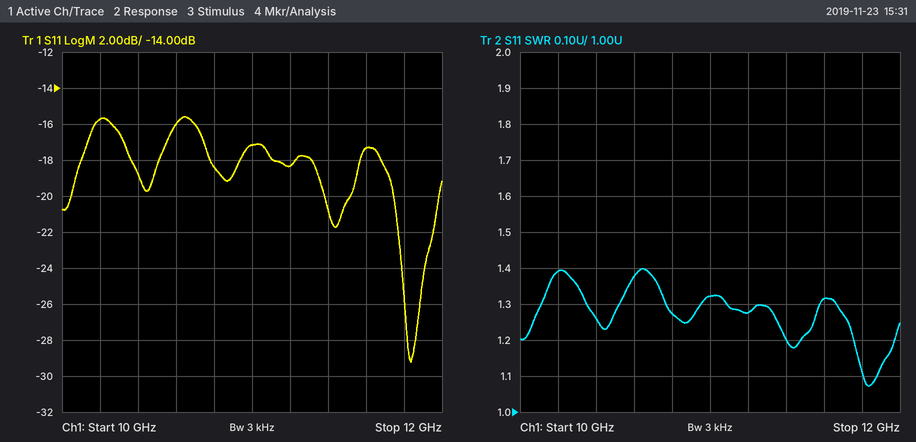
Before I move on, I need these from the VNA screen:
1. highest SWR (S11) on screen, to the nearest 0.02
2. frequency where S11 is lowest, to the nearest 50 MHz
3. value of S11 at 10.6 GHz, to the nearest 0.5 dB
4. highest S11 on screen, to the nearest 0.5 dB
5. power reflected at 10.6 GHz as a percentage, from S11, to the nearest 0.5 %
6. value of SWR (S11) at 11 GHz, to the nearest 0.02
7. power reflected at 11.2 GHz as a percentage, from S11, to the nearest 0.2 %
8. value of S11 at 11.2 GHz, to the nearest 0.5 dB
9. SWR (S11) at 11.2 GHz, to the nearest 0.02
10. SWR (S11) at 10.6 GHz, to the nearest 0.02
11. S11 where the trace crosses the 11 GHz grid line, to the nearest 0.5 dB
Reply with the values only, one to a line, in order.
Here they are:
1.40
11.85 GHz
-16.0 dB
-15.5 dB
2.5 %
1.32
1.4 %
-18.5 dB
1.28
1.38
-17.0 dB
